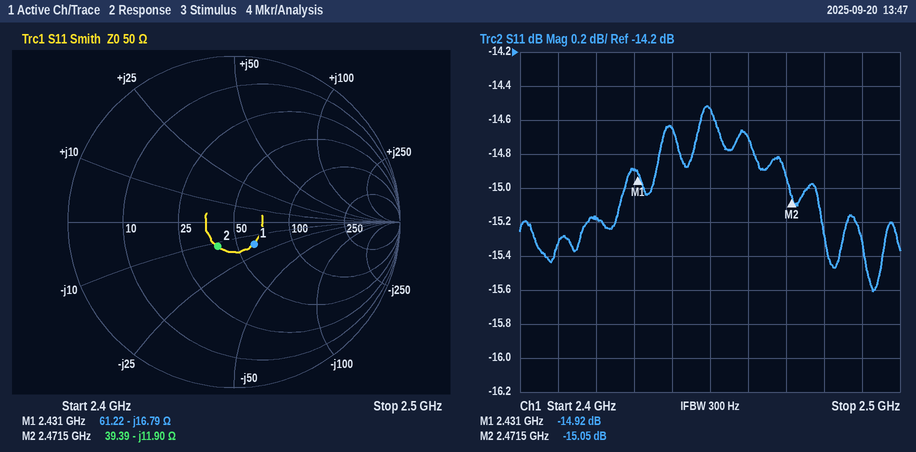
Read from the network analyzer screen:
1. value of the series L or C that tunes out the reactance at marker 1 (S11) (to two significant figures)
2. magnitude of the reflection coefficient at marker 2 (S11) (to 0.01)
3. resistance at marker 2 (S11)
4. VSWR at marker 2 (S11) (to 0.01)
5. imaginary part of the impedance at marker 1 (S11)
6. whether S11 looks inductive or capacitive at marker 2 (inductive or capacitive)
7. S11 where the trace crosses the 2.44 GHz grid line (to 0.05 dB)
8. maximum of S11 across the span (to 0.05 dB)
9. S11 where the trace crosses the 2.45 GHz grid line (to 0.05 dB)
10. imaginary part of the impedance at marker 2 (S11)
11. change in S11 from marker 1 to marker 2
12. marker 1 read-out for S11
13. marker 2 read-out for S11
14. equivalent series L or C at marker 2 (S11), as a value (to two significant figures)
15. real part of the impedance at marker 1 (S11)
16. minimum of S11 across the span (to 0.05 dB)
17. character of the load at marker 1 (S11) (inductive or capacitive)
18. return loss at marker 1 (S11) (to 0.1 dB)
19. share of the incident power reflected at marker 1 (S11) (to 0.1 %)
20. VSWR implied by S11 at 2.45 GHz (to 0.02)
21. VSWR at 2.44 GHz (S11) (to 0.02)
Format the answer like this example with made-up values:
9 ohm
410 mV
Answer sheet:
1.1 nH
0.18
39.39 Ω
1.43
-16.79 Ω
capacitive
-14.65 dB
-14.50 dB
-14.55 dB
-11.90 Ω
-0.13 dB
-14.92 dB
-15.05 dB
5.4 pF
61.22 Ω
-15.60 dB
capacitive
14.9 dB
3.2 %
1.46
1.46
